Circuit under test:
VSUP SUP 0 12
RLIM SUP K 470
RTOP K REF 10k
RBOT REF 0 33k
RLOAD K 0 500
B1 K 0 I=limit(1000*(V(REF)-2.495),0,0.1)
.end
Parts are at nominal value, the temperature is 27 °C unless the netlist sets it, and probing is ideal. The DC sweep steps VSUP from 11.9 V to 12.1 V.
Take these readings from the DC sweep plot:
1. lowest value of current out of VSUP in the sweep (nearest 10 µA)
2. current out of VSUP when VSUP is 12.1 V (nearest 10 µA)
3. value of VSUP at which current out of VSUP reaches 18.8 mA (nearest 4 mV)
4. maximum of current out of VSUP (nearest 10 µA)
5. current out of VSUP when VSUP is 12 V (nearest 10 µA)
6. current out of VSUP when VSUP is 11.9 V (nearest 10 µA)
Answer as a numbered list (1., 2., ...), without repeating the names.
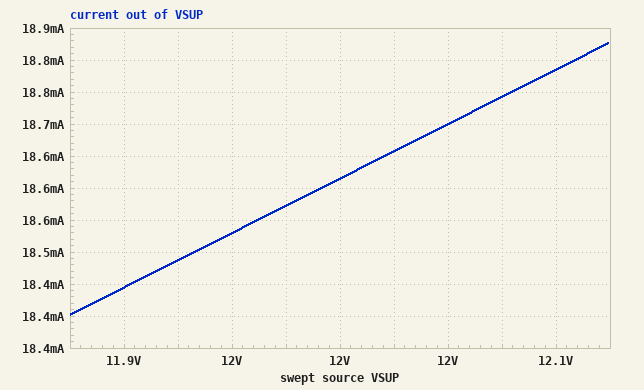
1. 18.40 mA
2. 18.74 mA
3. 12.064 V
4. 18.83 mA
5. 18.57 mA
6. 18.49 mA
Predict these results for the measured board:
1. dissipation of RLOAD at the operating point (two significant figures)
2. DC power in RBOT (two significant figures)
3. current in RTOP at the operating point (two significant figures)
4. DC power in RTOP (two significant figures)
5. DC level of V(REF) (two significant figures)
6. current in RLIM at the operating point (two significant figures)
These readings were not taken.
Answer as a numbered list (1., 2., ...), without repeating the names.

1. 21 mW
2. 190 µW
3. 76 µA
4. 57 µW
5. 2.5 V
6. 19 mA
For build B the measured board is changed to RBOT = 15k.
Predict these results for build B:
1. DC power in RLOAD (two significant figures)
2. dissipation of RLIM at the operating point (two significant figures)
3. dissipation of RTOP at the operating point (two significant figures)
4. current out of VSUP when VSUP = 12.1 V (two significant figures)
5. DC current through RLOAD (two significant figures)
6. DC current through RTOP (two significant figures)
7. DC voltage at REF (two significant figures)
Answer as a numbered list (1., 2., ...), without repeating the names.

1. 35 mW
2. 130 mW
3. 280 µW
4. 17 mA
5. 8.3 mA
6. 170 µA
7. 2.5 V
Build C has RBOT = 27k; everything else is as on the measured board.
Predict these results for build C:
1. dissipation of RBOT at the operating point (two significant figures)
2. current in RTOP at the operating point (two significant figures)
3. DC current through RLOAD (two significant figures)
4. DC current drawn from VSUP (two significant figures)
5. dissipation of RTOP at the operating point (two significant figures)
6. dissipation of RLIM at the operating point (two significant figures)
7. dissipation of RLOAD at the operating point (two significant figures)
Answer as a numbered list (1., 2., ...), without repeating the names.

1. 230 µW
2. 92 µA
3. 6.8 mA
4. 18 mA
5. 85 µW
6. 160 mW
7. 23 mW
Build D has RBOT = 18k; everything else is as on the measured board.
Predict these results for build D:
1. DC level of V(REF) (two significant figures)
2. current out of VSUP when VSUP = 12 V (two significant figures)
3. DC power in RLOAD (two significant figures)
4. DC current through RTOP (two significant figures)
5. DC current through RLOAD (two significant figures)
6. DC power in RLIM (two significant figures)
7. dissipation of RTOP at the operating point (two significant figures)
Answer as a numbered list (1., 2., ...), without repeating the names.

1. 2.5 V
2. 17 mA
3. 30 mW
4. 140 µA
5. 7.8 mA
6. 140 mW
7. 190 µW
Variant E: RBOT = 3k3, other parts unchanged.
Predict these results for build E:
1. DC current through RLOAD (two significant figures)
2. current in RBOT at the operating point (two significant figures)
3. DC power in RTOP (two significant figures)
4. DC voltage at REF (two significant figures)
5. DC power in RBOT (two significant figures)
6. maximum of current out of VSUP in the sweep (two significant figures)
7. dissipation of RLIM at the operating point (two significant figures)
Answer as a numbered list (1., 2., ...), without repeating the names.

1. 12 mA
2. 460 µA
3. 2.1 mW
4. 1.5 V
5. 690 µW
6. 13 mA
7. 75 mW
